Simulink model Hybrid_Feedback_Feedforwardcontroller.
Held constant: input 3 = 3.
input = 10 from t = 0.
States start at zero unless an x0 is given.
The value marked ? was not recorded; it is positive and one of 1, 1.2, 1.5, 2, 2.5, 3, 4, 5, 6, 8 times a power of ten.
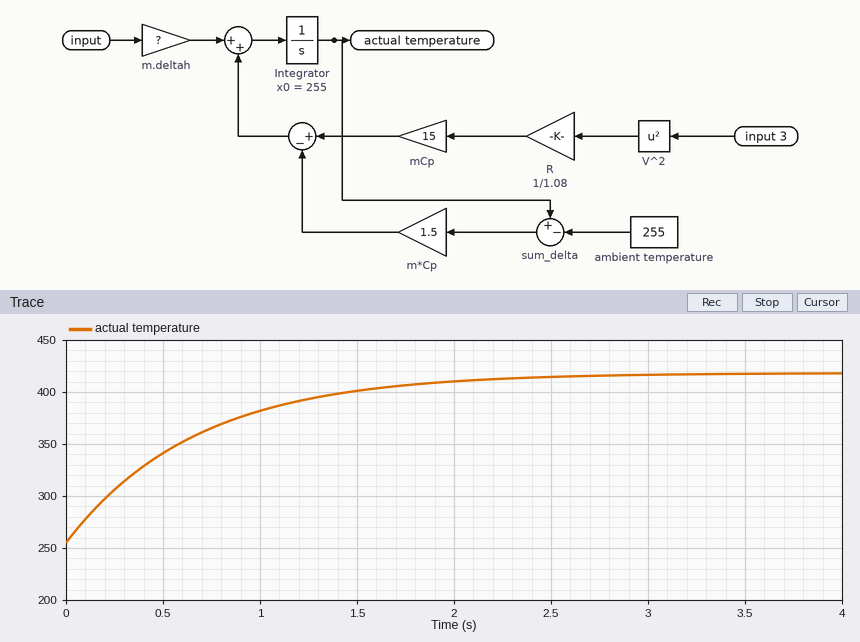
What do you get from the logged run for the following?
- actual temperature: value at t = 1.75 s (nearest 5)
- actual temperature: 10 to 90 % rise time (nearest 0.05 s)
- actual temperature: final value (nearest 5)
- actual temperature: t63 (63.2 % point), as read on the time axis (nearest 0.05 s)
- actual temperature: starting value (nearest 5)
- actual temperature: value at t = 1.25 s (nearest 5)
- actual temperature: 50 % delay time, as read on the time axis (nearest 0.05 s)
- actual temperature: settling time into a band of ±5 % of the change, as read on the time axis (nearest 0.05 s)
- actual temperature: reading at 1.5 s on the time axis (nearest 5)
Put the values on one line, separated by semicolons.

405; 1.45 s; 420; 0.65 s; 255; 395; 0.45 s; 2.00 s; 400
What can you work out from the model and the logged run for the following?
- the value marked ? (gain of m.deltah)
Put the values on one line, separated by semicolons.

12
